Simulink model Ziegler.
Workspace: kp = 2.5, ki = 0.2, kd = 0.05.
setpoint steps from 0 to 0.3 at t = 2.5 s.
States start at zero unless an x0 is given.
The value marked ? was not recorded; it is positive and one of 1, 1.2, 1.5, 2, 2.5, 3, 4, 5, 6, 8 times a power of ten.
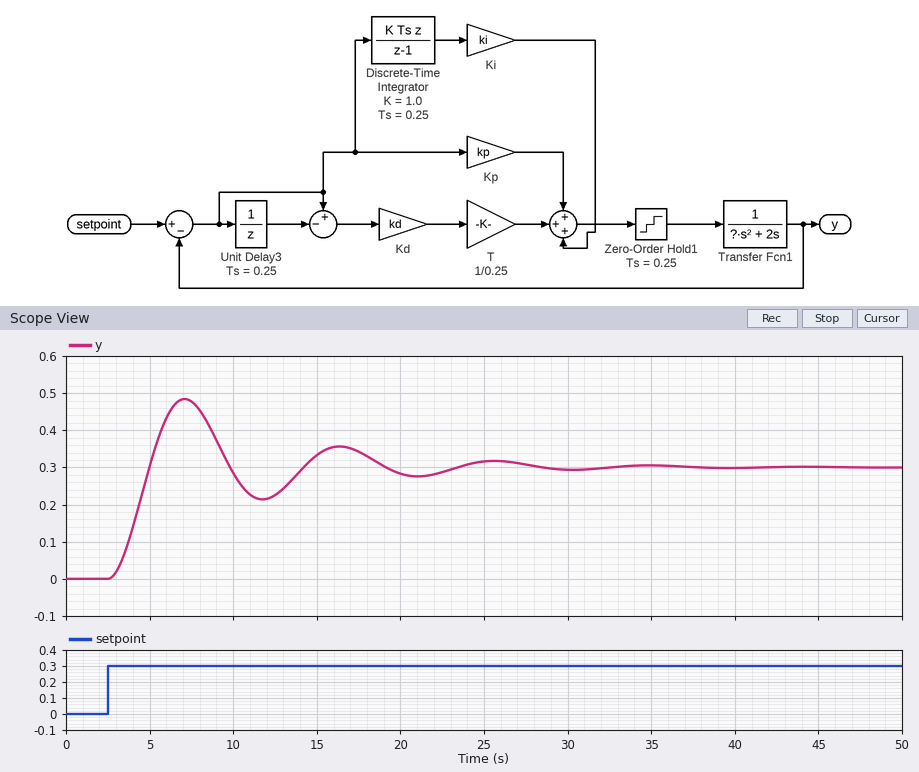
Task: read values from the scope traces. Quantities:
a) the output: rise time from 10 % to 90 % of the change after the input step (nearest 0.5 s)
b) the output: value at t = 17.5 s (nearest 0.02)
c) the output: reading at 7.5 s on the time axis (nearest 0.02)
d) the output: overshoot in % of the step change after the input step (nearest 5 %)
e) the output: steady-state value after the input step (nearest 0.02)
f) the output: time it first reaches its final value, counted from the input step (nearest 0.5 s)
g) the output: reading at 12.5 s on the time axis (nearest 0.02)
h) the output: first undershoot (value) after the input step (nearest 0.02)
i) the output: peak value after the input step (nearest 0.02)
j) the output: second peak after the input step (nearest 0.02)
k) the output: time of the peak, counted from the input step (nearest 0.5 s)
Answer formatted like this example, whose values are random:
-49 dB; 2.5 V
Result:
1.5 s; 0.34; 0.48; 60 %; 0.30; 2.5 s; 0.22; 0.22; 0.48; 0.36; 4.5 s
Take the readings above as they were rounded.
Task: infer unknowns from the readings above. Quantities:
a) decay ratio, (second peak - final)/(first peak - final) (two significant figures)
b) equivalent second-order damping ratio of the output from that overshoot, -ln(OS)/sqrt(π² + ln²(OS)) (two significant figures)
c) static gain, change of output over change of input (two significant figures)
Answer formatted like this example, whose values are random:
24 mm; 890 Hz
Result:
0.33; 0.16; 1.0
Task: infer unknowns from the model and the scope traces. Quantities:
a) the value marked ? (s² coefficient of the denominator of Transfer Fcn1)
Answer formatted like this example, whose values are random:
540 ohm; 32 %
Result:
5
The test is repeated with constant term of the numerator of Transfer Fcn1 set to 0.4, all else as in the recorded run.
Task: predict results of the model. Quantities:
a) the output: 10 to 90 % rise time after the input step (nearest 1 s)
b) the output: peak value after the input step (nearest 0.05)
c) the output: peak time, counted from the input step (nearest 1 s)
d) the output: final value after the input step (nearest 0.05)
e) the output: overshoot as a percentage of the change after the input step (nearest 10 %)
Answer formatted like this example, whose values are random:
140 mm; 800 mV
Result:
3 s; 0.45; 8 s; 0.30; 50 %
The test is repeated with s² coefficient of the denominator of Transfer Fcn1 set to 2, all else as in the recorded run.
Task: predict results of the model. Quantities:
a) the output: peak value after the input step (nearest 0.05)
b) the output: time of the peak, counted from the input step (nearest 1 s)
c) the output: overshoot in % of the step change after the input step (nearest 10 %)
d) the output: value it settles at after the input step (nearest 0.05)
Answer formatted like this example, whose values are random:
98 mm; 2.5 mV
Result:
0.40; 3 s; 40 %; 0.30
